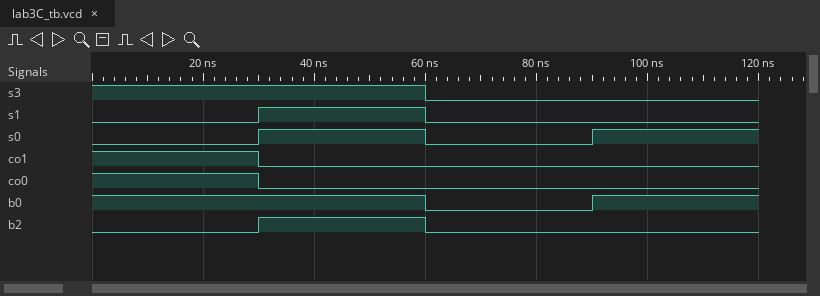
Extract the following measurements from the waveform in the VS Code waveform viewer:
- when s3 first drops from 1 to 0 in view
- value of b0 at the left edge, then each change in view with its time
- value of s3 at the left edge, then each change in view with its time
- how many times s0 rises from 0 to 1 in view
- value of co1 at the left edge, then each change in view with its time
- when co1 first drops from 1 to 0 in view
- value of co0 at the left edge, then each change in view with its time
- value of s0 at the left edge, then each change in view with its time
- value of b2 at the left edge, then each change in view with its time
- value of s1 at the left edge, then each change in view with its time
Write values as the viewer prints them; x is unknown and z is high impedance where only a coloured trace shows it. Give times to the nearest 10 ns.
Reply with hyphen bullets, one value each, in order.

- 60 ns
- 1, 0 at 60 ns, 1 at 90 ns
- 1, 0 at 60 ns
- 2
- 1, 0 at 30 ns
- 30 ns
- 1, 0 at 30 ns
- 0, 1 at 30 ns, 0 at 60 ns, 1 at 90 ns
- 0, 1 at 30 ns, 0 at 60 ns
- 0, 1 at 30 ns, 0 at 60 ns
